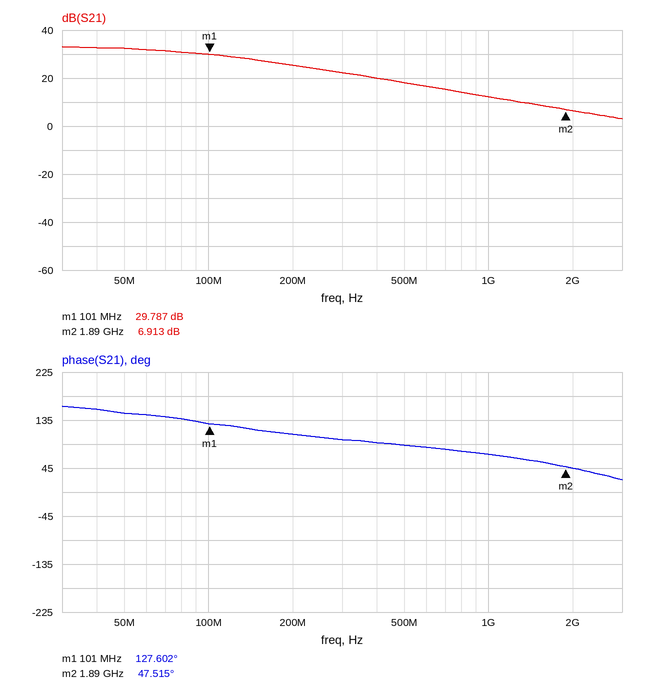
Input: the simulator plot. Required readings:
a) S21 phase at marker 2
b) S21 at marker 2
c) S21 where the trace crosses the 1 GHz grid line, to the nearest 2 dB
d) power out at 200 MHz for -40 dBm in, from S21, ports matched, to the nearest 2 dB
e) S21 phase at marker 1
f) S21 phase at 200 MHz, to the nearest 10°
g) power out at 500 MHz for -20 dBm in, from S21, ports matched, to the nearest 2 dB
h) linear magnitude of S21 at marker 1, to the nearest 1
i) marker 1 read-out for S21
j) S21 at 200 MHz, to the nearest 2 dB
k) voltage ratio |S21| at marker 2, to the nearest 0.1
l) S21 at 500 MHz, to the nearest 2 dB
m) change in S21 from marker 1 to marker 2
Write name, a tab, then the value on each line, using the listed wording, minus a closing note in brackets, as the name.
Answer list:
S21 phase at marker 2	47.515°
S21 at marker 2	6.913 dB
S21 where the trace crosses the 1 GHz grid line, to the nearest 2 dB	12 dB
power out at 200 MHz for -40 dBm in, from S21, ports matched, to the nearest 2 dB	-14 dBm
S21 phase at marker 1	127.602°
S21 phase at 200 MHz, to the nearest 10°	110°
power out at 500 MHz for -20 dBm in, from S21, ports matched, to the nearest 2 dB	-2 dBm
linear magnitude of S21 at marker 1, to the nearest 1	31
marker 1 read-out for S21	29.787 dB
S21 at 200 MHz, to the nearest 2 dB	26 dB
voltage ratio |S21| at marker 2, to the nearest 0.1	2.2
S21 at 500 MHz, to the nearest 2 dB	18 dB
change in S21 from marker 1 to marker 2	-22.874 dB
